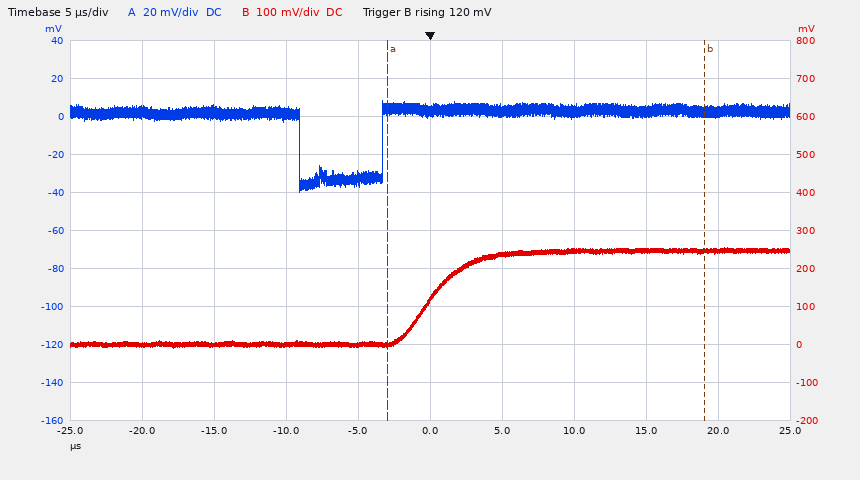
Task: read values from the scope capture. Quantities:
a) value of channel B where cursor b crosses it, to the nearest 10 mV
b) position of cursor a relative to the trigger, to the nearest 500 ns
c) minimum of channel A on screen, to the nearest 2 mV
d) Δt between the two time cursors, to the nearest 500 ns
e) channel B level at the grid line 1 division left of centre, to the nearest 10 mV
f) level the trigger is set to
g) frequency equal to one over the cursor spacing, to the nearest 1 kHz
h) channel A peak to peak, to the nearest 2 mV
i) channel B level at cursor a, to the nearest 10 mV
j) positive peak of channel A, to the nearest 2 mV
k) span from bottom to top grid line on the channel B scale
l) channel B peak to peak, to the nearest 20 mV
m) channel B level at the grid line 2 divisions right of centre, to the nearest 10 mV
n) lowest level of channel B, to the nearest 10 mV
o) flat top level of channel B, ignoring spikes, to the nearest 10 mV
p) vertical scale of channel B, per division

250 mV
-3.0 µs
-40 mV
22.0 µs
0 mV
120 mV
45 kHz
48 mV
0 mV
8 mV
1 V
260 mV
250 mV
-10 mV
250 mV
100 mV
